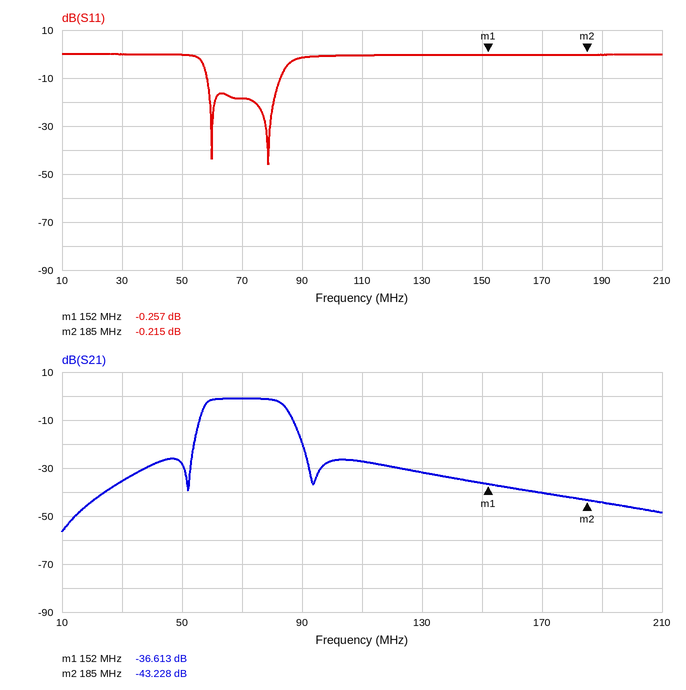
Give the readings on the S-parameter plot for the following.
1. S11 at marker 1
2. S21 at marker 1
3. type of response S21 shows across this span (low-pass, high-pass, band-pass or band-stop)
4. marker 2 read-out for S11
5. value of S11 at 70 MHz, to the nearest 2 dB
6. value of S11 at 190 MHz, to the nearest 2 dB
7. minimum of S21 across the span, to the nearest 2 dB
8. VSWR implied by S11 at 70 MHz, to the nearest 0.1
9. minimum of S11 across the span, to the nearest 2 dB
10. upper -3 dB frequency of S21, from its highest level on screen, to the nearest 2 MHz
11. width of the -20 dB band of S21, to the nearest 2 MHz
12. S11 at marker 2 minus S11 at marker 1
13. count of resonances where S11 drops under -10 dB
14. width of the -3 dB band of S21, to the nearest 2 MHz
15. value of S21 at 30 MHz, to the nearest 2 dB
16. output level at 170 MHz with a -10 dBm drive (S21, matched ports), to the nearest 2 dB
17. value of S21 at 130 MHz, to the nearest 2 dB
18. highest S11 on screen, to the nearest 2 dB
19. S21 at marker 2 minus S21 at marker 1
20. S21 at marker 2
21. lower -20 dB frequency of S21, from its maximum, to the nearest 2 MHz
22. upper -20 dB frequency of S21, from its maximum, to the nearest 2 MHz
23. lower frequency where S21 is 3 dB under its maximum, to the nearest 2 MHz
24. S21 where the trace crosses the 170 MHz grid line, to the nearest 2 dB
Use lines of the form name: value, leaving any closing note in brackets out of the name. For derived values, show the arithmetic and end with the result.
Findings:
S11 at marker 1: -0.257 dB
S21 at marker 1: -36.613 dB
type of response S21 shows across this span: band-pass
marker 2 read-out for S11: -0.215 dB
value of S11 at 70 MHz, to the nearest 2 dB: -18 dB
value of S11 at 190 MHz, to the nearest 2 dB: 0 dB
minimum of S21 across the span, to the nearest 2 dB: -56 dB
VSWR implied by S11 at 70 MHz, to the nearest 0.1: |Γ| = 10^(-18/20) = 0.1259; VSWR = (1 + 0.1259)/(1 − 0.1259) ≈ 1.3
minimum of S11 across the span, to the nearest 2 dB: -46 dB
upper -3 dB frequency of S21, from its highest level on screen, to the nearest 2 MHz: 84 MHz
width of the -20 dB band of S21, to the nearest 2 MHz: 90 MHz − 54 MHz = 36 MHz
S11 at marker 2 minus S11 at marker 1: -0.215 − (-0.257) = 0.042 dB
count of resonances where S11 drops under -10 dB: 2
width of the -3 dB band of S21, to the nearest 2 MHz: 84 MHz − 58 MHz = 26 MHz
value of S21 at 30 MHz, to the nearest 2 dB: -36 dB
output level at 170 MHz with a -10 dBm drive (S21, matched ports), to the nearest 2 dB: -10 dBm + (-40 dB) = -50 dBm
value of S21 at 130 MHz, to the nearest 2 dB: -32 dB
highest S11 on screen, to the nearest 2 dB: 0 dB
S21 at marker 2 minus S21 at marker 1: -43.228 − (-36.613) = -6.615 dB
S21 at marker 2: -43.228 dB
lower -20 dB frequency of S21, from its maximum, to the nearest 2 MHz: 54 MHz
upper -20 dB frequency of S21, from its maximum, to the nearest 2 MHz: 90 MHz
lower frequency where S21 is 3 dB under its maximum, to the nearest 2 MHz: 58 MHz
S21 where the trace crosses the 170 MHz grid line, to the nearest 2 dB: -40 dB
